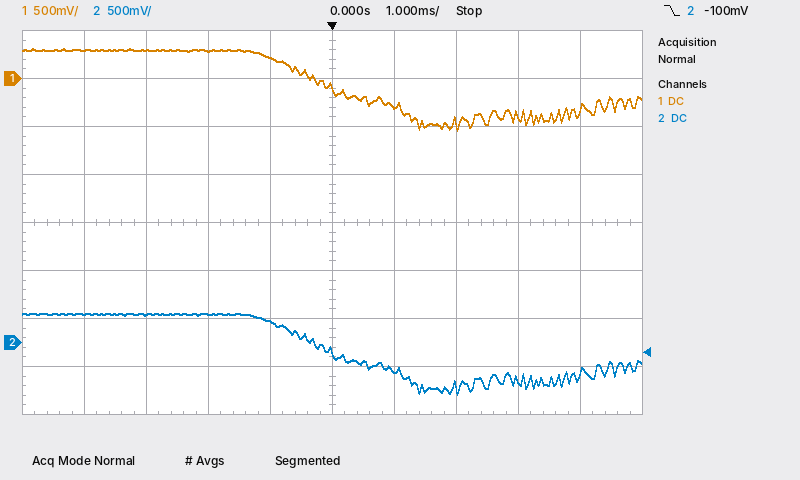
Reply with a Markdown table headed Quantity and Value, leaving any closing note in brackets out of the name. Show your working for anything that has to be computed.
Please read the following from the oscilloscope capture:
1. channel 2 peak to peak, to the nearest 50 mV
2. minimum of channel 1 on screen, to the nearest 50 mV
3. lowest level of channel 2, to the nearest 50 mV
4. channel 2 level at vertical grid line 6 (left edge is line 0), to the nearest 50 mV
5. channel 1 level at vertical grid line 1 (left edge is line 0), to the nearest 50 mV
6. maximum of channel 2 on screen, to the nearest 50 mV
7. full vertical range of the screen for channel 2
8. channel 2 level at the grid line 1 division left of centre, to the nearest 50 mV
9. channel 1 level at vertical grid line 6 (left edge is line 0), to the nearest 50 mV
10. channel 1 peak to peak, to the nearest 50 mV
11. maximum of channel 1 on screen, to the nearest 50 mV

| Quantity | Value |
|---|---|
| channel 2 peak to peak, to the nearest 50 mV | 300 mV − (-550 mV) = 850 mV |
| minimum of channel 1 on screen, to the nearest 50 mV | -550 mV |
| lowest level of channel 2, to the nearest 50 mV | -550 mV |
| channel 2 level at vertical grid line 6 (left edge is line 0), to the nearest 50 mV | -300 mV |
| channel 1 level at vertical grid line 1 (left edge is line 0), to the nearest 50 mV | 300 mV |
| maximum of channel 2 on screen, to the nearest 50 mV | 300 mV |
| full vertical range of the screen for channel 2 | 4 V |
| channel 2 level at the grid line 1 division left of centre, to the nearest 50 mV | 200 mV |
| channel 1 level at vertical grid line 6 (left edge is line 0), to the nearest 50 mV | -300 mV |
| channel 1 peak to peak, to the nearest 50 mV | 300 mV − (-550 mV) = 850 mV |
| maximum of channel 1 on screen, to the nearest 50 mV | 300 mV |
